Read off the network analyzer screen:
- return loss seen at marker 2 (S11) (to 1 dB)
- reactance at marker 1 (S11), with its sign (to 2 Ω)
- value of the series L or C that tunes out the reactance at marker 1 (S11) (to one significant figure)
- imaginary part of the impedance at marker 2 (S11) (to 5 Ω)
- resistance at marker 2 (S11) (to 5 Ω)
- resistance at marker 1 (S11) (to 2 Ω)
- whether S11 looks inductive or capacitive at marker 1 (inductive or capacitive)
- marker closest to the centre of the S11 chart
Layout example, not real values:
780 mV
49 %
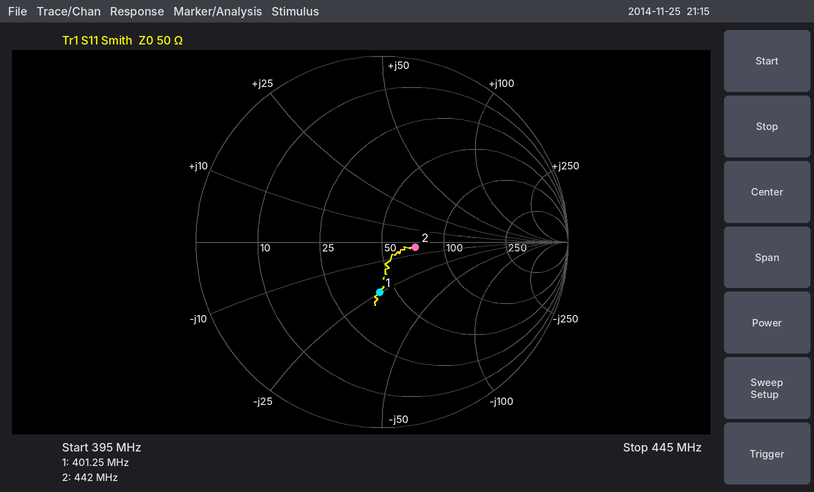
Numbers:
15 dB
-24 Ω
10 nH
-5 Ω
70 Ω
42 Ω
capacitive
marker 2
